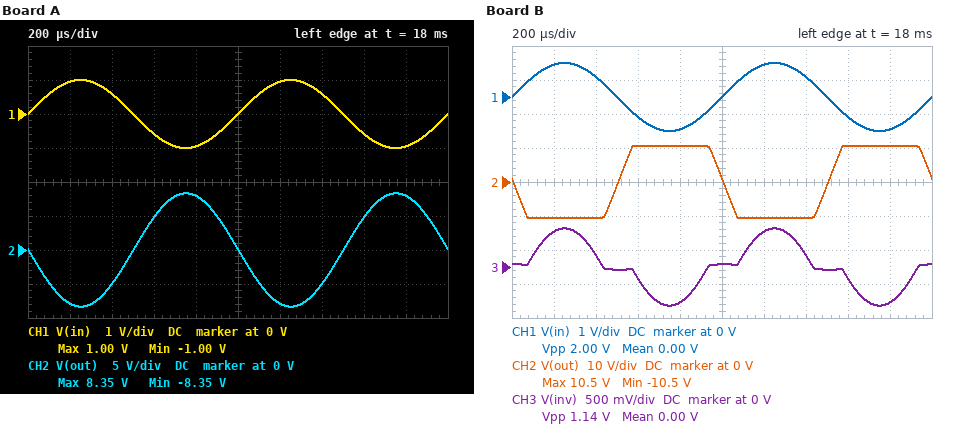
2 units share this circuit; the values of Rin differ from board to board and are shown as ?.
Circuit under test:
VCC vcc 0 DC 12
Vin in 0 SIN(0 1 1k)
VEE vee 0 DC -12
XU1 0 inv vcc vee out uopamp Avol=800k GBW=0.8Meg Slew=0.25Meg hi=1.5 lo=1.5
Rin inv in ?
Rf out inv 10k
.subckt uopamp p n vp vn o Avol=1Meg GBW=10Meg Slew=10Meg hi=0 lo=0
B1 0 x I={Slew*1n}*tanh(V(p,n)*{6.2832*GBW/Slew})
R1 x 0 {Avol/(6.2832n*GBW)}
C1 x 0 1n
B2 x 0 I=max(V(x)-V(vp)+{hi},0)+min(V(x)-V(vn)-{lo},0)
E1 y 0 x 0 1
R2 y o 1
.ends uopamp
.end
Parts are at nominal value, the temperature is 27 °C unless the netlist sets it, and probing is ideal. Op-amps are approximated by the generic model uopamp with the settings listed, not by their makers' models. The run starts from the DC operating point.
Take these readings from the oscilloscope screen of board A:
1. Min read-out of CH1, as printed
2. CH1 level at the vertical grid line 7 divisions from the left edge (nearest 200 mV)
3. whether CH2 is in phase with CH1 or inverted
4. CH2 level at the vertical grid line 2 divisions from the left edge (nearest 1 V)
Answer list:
-1.00 V
600 mV
inverted
-5 V
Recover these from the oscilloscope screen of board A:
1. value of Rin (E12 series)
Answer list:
1.2 kΩ
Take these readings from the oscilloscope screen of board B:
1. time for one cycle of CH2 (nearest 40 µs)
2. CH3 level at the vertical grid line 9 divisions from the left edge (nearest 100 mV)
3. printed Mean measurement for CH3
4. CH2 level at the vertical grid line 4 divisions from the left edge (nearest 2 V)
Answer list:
1.00 ms
-500 mV
0.00 V
10 V
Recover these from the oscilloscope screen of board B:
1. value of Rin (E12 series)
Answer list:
390 Ω
